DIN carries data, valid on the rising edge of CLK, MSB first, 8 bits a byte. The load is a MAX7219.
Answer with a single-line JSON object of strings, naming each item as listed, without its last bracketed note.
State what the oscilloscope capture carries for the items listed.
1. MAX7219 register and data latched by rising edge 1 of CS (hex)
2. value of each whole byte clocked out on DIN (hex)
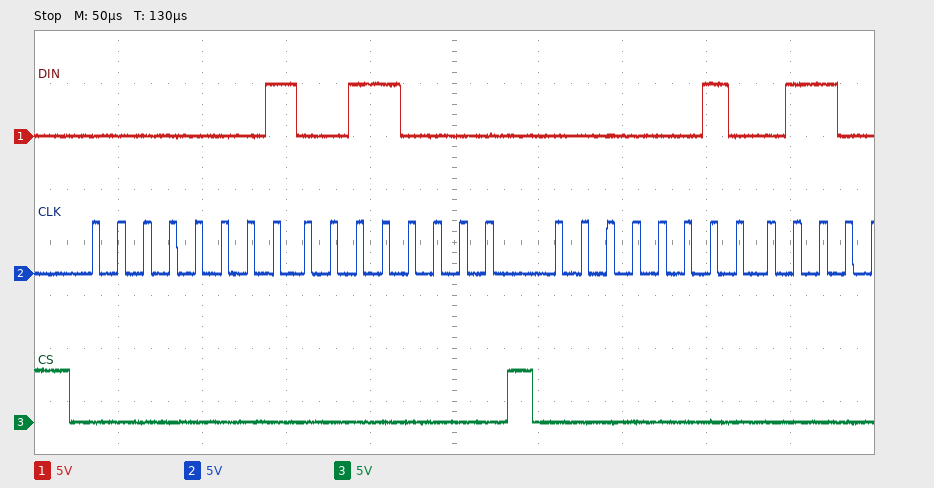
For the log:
{"MAX7219 register and data latched by rising edge 1 of CS": "register 0x1, data 0x30", "value of each whole byte clocked out on DIN": "0x01 0x30 0x02"}
